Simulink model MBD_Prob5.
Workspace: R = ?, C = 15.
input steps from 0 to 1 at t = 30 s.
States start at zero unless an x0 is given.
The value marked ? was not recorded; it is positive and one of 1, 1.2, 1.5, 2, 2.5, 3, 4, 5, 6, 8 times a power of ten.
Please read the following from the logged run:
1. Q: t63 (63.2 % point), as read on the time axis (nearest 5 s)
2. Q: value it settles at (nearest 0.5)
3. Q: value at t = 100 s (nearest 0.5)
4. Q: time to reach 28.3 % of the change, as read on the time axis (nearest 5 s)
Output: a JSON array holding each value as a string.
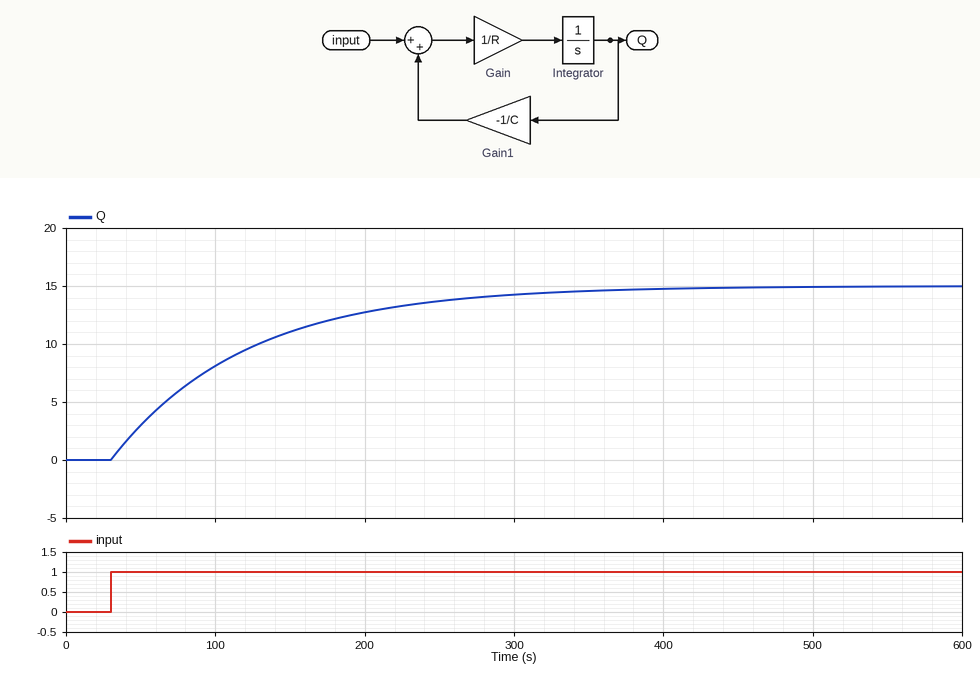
["120 s", "15.0", "8.0", "60 s"]
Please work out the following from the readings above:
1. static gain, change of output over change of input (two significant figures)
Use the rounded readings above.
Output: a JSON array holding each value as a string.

["15"]
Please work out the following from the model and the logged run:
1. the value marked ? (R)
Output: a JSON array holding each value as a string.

["6"]
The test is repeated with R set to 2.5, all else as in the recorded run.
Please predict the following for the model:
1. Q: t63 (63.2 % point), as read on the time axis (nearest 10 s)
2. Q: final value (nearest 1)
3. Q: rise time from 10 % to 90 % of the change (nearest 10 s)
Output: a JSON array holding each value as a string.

["70 s", "15", "80 s"]
